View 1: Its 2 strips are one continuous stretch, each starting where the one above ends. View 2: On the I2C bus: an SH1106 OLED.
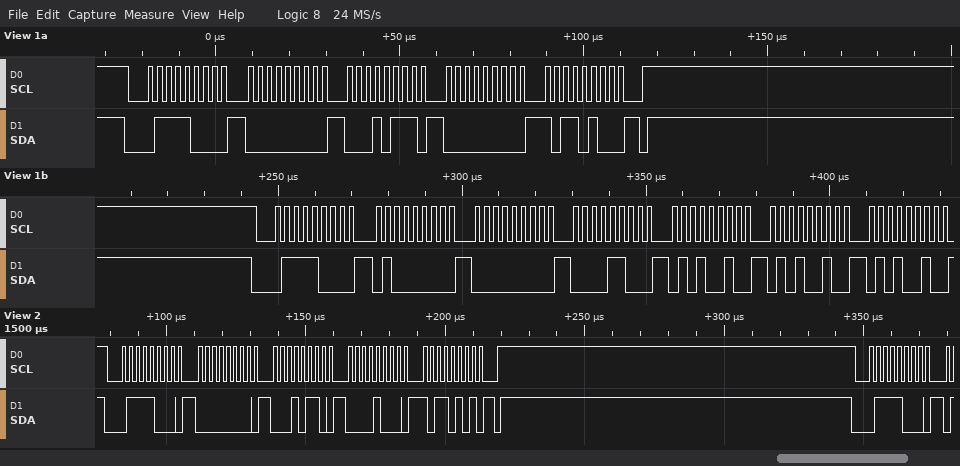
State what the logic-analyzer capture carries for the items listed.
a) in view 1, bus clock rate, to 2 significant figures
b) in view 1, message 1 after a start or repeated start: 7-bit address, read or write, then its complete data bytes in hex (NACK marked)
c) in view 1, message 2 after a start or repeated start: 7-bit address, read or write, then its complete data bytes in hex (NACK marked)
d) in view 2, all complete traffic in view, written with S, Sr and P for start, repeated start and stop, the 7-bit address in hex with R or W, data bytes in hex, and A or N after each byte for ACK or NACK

400 kHz
0x3C write: 00 17 00 B4
0x3C write: 40 00 0C 52 52 52
S 3CW A 00 A 16 A 08 A B5 A P S 3CW A
